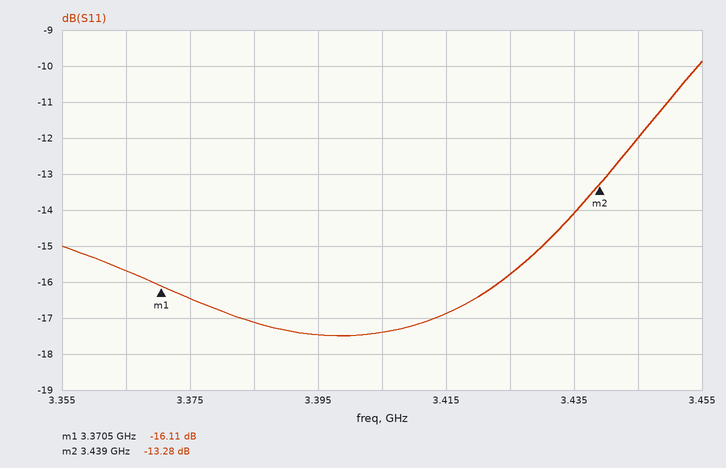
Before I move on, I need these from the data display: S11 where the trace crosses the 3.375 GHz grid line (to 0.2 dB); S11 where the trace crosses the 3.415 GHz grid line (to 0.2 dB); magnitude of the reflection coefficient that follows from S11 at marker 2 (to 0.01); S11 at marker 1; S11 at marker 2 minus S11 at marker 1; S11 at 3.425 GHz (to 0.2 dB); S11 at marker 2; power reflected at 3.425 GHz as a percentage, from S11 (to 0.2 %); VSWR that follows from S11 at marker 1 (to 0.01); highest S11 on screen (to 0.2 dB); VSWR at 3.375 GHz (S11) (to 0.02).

-16.4 dB
-16.8 dB
0.22
-16.11 dB
2.83 dB
-15.8 dB
-13.28 dB
2.6 %
1.37
-9.8 dB
1.36
